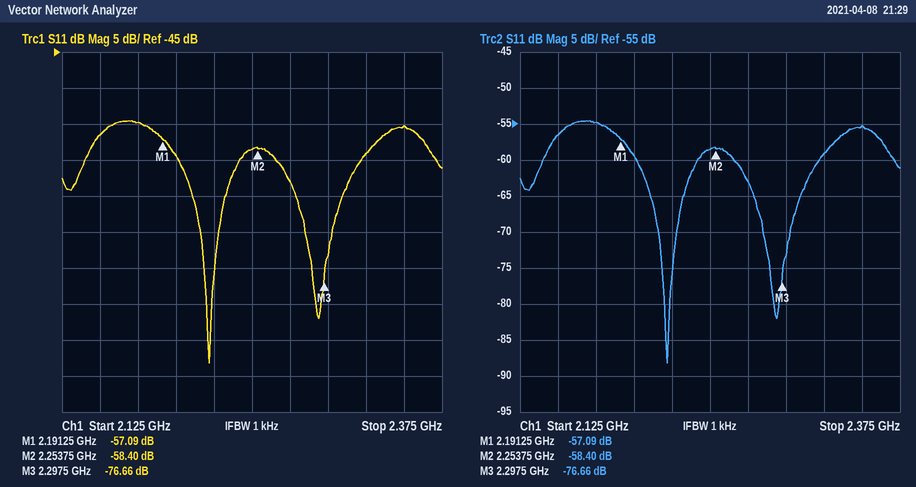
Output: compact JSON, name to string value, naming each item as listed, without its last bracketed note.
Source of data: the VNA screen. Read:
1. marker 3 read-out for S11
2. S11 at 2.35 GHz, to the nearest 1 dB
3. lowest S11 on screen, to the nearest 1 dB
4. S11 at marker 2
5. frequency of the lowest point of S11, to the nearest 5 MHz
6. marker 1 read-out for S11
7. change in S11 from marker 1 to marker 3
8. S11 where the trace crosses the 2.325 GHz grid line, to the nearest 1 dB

{"marker 3 read-out for S11": "-76.66 dB", "S11 at 2.35 GHz, to the nearest 1 dB": "-55 dB", "lowest S11 on screen, to the nearest 1 dB": "-88 dB", "S11 at marker 2": "-58.40 dB", "frequency of the lowest point of S11, to the nearest 5 MHz": "2.220 GHz", "marker 1 read-out for S11": "-57.09 dB", "change in S11 from marker 1 to marker 3": "-19.57 dB", "S11 where the trace crosses the 2.325 GHz grid line, to the nearest 1 dB": "-59 dB"}
